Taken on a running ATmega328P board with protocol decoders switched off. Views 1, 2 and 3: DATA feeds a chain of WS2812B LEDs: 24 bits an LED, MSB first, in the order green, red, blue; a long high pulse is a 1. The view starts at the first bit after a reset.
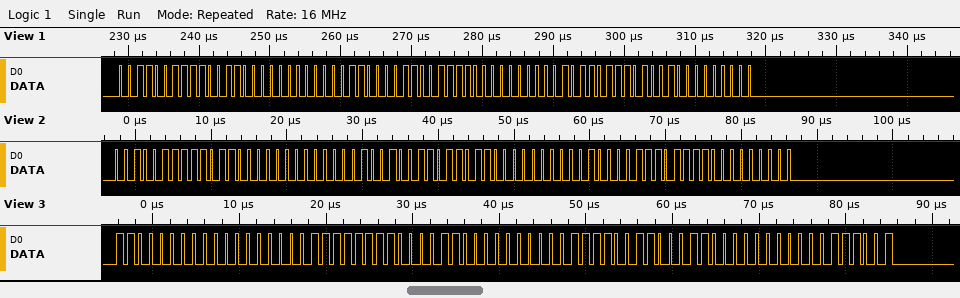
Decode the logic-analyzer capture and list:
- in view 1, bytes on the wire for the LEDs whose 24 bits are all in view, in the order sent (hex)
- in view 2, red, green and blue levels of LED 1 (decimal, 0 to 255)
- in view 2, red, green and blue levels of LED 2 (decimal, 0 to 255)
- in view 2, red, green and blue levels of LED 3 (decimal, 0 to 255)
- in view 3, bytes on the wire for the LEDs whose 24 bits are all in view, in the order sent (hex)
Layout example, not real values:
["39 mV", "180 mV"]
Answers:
["33 CC 00 30 CF 00 2D D2 00", "216, 39, 0", "219, 36, 0", "222, 33, 0", "C0 00 3F C3 00 3C C6 00 39"]
